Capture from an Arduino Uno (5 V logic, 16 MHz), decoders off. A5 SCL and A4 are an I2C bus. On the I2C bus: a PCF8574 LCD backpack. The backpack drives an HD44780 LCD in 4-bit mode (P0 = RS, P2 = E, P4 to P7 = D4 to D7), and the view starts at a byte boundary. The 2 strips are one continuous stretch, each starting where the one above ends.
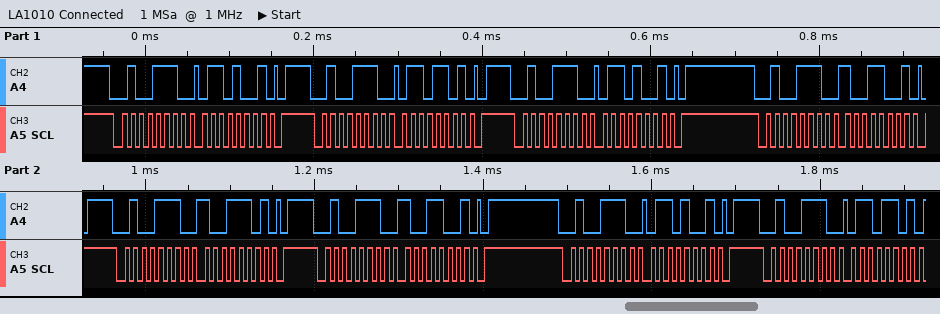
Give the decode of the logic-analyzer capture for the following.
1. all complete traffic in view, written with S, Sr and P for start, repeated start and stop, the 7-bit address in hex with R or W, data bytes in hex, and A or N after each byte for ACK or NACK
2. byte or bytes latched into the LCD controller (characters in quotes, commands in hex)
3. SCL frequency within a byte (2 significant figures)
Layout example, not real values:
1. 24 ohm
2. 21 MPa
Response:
1. S 27W A 69 A P S 27W A 6D A P S 27W A 69 A P S 27W A 99 A P S 27W A 9D A P S 27W A 99 A P S 27W A 69 A P S 27W A 6D A
2. 'i'
3. 100 kHz
